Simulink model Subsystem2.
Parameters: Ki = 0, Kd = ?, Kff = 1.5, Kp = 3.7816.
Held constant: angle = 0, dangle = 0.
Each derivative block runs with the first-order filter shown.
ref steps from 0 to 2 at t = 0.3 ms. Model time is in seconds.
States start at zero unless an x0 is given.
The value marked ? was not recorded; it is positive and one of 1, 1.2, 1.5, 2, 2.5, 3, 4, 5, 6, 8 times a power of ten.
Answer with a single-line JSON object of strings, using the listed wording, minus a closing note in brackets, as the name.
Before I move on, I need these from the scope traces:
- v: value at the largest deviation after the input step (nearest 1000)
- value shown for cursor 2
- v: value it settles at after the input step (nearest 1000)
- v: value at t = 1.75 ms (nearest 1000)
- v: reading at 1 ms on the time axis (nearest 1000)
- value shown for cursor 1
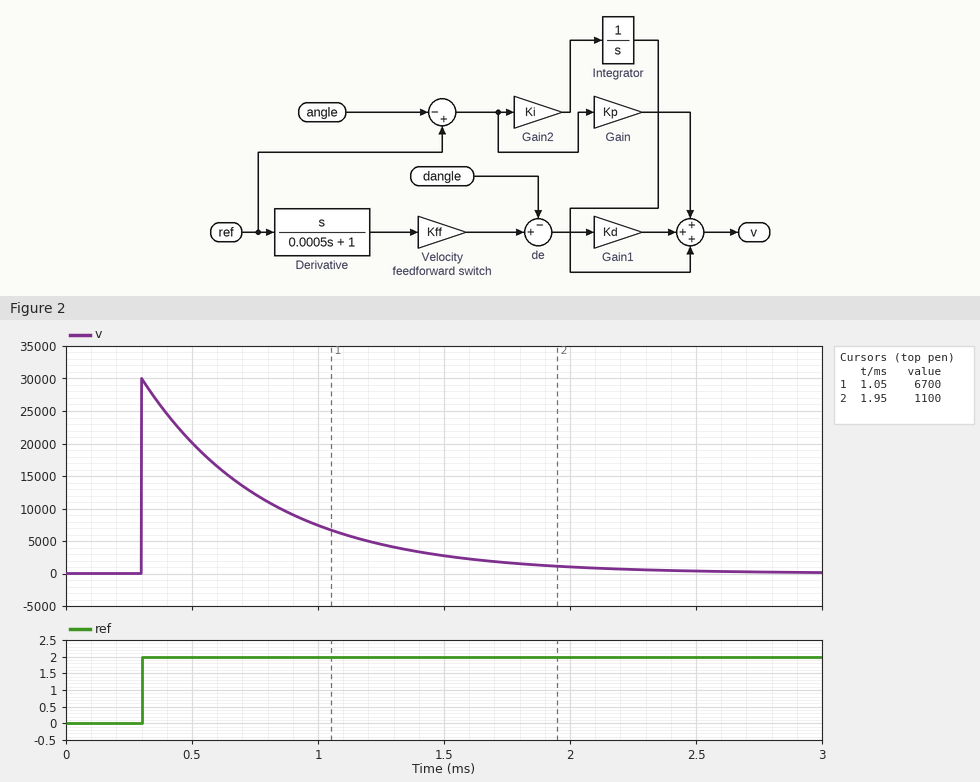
{"v: value at the largest deviation after the input step": "30000", "value shown for cursor 2": "1100", "v: value it settles at after the input step": "0", "v: value at t = 1.75 ms": "2000", "v: reading at 1 ms on the time axis": "7000", "value shown for cursor 1": "6700"}
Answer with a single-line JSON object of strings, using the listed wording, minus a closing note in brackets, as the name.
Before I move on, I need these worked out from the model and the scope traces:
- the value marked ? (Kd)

{"the value marked ?": "5"}
